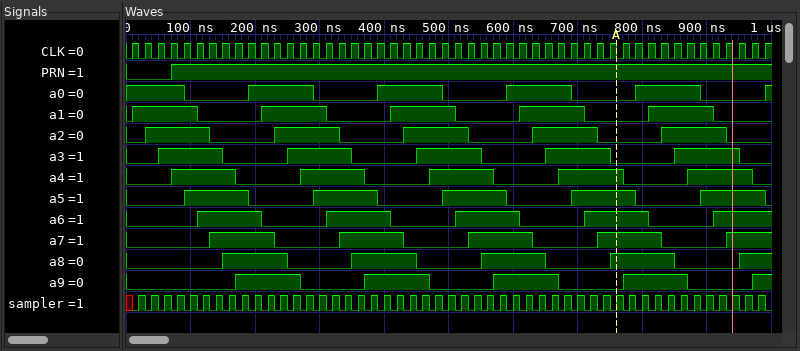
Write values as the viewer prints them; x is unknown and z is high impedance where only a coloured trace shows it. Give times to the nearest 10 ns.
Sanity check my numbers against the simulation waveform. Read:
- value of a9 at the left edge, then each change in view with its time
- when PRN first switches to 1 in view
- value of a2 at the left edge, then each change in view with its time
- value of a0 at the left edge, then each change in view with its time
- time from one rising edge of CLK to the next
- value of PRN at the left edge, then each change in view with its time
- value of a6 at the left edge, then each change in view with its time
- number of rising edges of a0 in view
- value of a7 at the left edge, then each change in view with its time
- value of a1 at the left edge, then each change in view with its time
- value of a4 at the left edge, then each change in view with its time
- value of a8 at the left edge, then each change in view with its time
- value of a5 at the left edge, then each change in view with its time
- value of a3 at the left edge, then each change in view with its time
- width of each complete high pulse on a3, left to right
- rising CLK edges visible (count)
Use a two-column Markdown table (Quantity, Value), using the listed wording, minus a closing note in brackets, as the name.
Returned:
| Quantity | Value |
|---|---|
| value of a9 at the left edge, then each change in view with its time | 0, 1 at 170 ns, 0 at 270 ns, 1 at 370 ns, 0 at 470 ns, 1 at 570 ns, 0 at 670 ns, 1 at 770 ns, 0 at 870 ns, 1 at 970 ns |
| when PRN first switches to 1 in view | 70 ns |
| value of a2 at the left edge, then each change in view with its time | 0, 1 at 30 ns, 0 at 130 ns, 1 at 230 ns, 0 at 330 ns, 1 at 430 ns, 0 at 530 ns, 1 at 630 ns, 0 at 730 ns, 1 at 830 ns, 0 at 930 ns |
| value of a0 at the left edge, then each change in view with its time | 1, 0 at 90 ns, 1 at 190 ns, 0 at 290 ns, 1 at 390 ns, 0 at 490 ns, 1 at 590 ns, 0 at 690 ns, 1 at 790 ns, 0 at 890 ns, 1 at 990 ns |
| time from one rising edge of CLK to the next | 20 ns |
| value of PRN at the left edge, then each change in view with its time | 0, 1 at 70 ns |
| value of a6 at the left edge, then each change in view with its time | 0, 1 at 110 ns, 0 at 210 ns, 1 at 310 ns, 0 at 410 ns, 1 at 510 ns, 0 at 610 ns, 1 at 710 ns, 0 at 810 ns, 1 at 910 ns |
| number of rising edges of a0 in view | 5 |
| value of a7 at the left edge, then each change in view with its time | 0, 1 at 130 ns, 0 at 230 ns, 1 at 330 ns, 0 at 430 ns, 1 at 530 ns, 0 at 630 ns, 1 at 730 ns, 0 at 830 ns, 1 at 930 ns |
| value of a1 at the left edge, then each change in view with its time | 0, 1 at 10 ns, 0 at 110 ns, 1 at 210 ns, 0 at 310 ns, 1 at 410 ns, 0 at 510 ns, 1 at 610 ns, 0 at 710 ns, 1 at 810 ns, 0 at 910 ns |
| value of a4 at the left edge, then each change in view with its time | 0, 1 at 70 ns, 0 at 170 ns, 1 at 270 ns, 0 at 370 ns, 1 at 470 ns, 0 at 570 ns, 1 at 670 ns, 0 at 770 ns, 1 at 870 ns, 0 at 970 ns |
| value of a8 at the left edge, then each change in view with its time | 0, 1 at 150 ns, 0 at 250 ns, 1 at 350 ns, 0 at 450 ns, 1 at 550 ns, 0 at 650 ns, 1 at 750 ns, 0 at 850 ns, 1 at 950 ns |
| value of a5 at the left edge, then each change in view with its time | 0, 1 at 90 ns, 0 at 190 ns, 1 at 290 ns, 0 at 390 ns, 1 at 490 ns, 0 at 590 ns, 1 at 690 ns, 0 at 790 ns, 1 at 890 ns, 0 at 990 ns |
| value of a3 at the left edge, then each change in view with its time | 0, 1 at 50 ns, 0 at 150 ns, 1 at 250 ns, 0 at 350 ns, 1 at 450 ns, 0 at 550 ns, 1 at 650 ns, 0 at 750 ns, 1 at 850 ns, 0 at 950 ns |
| width of each complete high pulse on a3, left to right | 100 ns, 100 ns, 100 ns, 100 ns, 100 ns |
| rising CLK edges visible | 50 |
